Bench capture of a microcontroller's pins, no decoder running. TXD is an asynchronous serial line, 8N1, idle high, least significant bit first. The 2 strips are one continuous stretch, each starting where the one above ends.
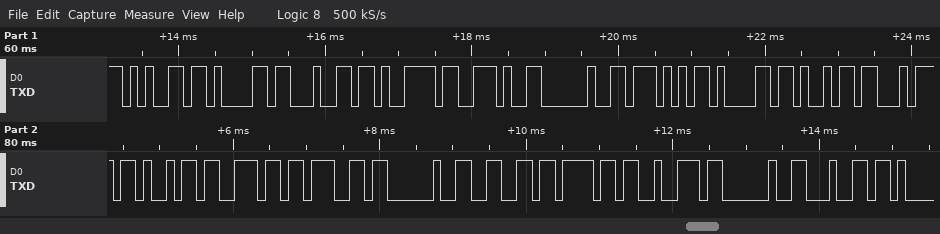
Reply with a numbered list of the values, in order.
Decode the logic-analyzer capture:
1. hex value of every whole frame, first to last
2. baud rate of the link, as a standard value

1. 0x65 0x61 0x64 0x79 0x2E 0x20 0x57 0x61 0x69 0x74 0x69 0x6E 0x67 0x20 0x66 0x6F 0x72 0x20 0x64
2. 9600 baud
